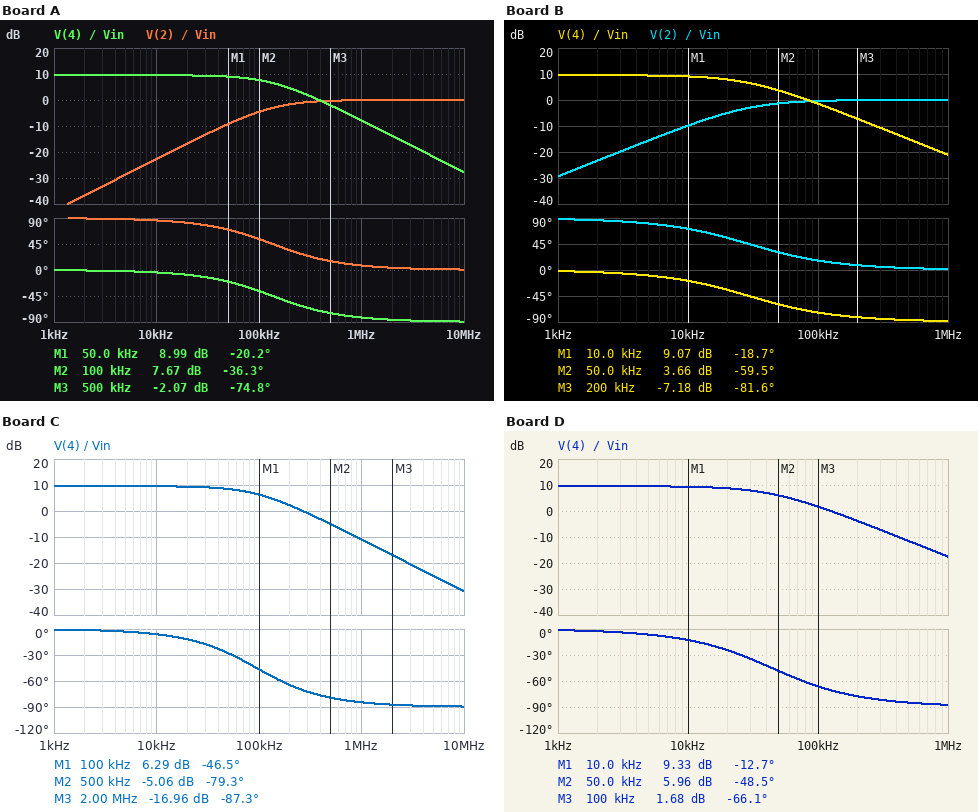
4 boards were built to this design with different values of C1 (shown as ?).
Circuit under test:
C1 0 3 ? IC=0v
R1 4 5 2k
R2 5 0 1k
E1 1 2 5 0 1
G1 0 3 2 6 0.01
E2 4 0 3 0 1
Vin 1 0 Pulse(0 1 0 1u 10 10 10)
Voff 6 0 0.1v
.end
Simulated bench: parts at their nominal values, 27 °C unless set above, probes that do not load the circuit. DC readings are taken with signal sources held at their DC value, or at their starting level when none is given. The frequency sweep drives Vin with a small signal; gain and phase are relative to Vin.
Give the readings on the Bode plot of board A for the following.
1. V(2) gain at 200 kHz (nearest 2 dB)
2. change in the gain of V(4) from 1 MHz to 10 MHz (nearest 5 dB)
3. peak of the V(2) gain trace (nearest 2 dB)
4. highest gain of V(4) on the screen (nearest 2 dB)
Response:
-2 dB
-20 dB
0 dB
10 dB
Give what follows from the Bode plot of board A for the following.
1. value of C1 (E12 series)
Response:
3.9 nF
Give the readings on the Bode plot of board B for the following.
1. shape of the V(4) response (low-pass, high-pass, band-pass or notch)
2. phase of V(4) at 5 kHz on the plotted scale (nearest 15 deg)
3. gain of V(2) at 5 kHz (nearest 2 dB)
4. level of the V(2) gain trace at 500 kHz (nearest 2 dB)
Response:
low-pass
-15 deg
-16 dB
0 dB
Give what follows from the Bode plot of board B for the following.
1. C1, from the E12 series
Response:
18 nF
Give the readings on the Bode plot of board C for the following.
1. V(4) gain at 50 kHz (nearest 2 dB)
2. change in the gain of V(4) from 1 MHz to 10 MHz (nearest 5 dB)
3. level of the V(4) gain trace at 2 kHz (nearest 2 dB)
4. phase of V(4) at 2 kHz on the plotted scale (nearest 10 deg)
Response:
8 dB
-20 dB
10 dB
0 deg
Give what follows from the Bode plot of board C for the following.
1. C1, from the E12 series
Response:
5.6 nF
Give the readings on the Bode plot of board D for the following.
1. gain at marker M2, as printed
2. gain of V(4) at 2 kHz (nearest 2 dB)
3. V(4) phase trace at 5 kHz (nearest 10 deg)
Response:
5.96 dB
10 dB
-10 deg
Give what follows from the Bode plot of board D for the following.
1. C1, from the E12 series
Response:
12 nF
